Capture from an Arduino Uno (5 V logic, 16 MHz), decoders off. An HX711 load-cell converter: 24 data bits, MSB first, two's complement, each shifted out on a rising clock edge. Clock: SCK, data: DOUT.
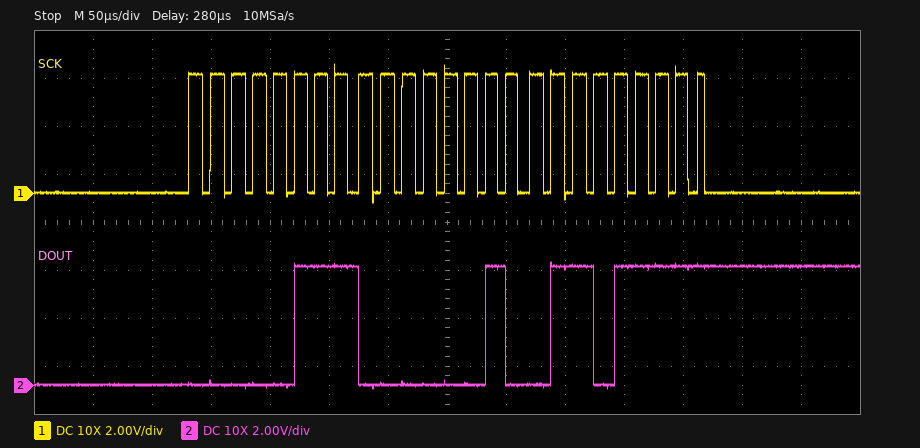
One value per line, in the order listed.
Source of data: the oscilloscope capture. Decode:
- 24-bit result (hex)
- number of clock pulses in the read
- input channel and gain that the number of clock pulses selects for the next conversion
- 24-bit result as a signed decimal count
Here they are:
0x07026F
25
channel A, gain 128
459375
